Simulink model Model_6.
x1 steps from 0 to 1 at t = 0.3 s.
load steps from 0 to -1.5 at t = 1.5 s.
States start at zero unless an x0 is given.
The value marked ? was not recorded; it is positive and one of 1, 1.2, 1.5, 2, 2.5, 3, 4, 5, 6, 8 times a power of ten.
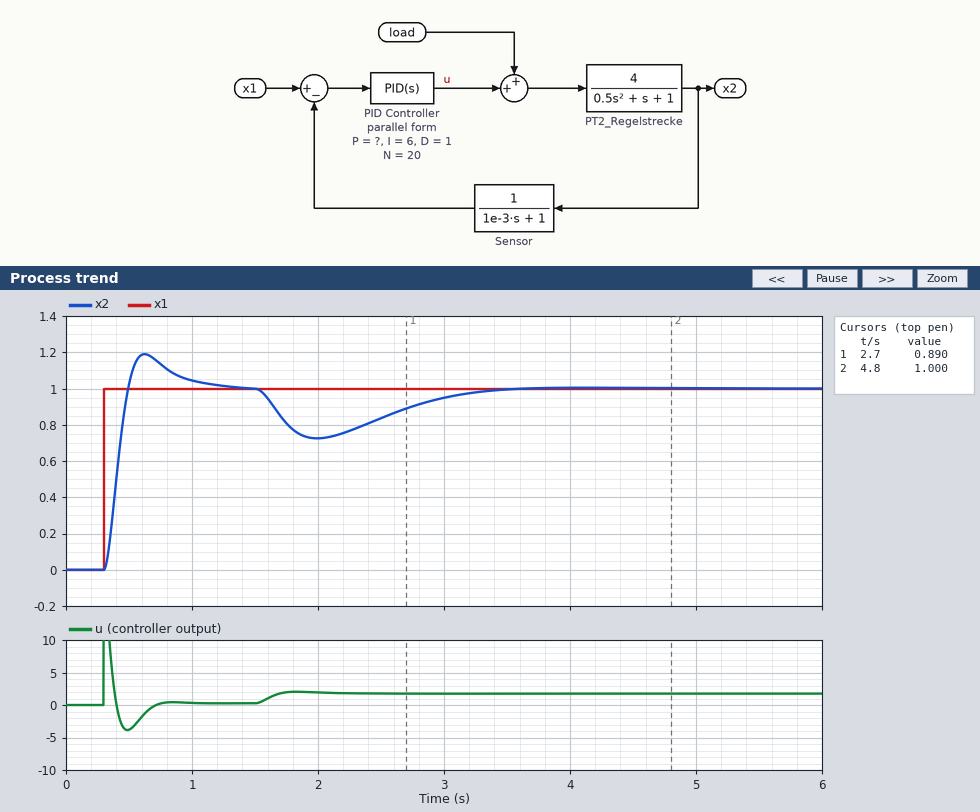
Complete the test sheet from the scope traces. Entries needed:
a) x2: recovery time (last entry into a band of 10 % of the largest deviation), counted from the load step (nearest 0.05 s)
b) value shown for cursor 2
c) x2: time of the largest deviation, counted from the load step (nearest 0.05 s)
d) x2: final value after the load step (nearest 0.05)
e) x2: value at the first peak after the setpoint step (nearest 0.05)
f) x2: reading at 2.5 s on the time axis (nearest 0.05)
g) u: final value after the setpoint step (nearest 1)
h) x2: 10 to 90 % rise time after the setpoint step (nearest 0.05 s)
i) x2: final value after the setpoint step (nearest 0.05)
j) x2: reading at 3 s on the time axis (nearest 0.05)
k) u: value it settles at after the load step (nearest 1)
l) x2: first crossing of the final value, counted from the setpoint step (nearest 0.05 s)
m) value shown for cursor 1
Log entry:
1.70 s
1.000
0.50 s
1.00
1.20
0.85
0
0.15 s
1.00
0.95
2
0.20 s
0.890
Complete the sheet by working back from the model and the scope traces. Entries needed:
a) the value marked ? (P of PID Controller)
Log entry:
4
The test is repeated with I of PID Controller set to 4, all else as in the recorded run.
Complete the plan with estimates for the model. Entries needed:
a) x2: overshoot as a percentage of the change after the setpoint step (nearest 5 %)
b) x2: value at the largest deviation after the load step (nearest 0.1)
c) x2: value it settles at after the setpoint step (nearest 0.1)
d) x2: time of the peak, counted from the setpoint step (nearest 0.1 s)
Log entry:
15 %
0.7
1.0
0.3 s
